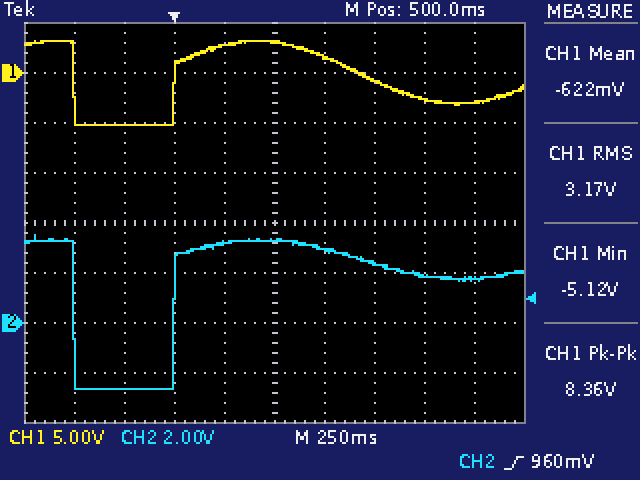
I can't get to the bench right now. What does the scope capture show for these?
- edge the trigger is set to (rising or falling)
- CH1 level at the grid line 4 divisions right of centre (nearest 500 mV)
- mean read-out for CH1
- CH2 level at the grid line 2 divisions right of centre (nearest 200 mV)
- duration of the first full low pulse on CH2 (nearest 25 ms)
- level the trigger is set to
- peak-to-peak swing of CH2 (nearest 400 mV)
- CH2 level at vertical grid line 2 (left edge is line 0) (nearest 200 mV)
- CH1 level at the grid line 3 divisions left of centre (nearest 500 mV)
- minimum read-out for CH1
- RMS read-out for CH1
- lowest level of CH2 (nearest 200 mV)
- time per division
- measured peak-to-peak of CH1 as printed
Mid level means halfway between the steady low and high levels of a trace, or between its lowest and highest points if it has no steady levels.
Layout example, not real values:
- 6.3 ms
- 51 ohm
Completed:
- rising
- -3.0 V
- -622 mV
- 2.4 V
- 500 ms
- 960 mV
- 6.0 V
- -2.6 V
- -5.0 V
- -5.12 V
- 3.17 V
- -2.6 V
- 250 ms
- 8.36 V
